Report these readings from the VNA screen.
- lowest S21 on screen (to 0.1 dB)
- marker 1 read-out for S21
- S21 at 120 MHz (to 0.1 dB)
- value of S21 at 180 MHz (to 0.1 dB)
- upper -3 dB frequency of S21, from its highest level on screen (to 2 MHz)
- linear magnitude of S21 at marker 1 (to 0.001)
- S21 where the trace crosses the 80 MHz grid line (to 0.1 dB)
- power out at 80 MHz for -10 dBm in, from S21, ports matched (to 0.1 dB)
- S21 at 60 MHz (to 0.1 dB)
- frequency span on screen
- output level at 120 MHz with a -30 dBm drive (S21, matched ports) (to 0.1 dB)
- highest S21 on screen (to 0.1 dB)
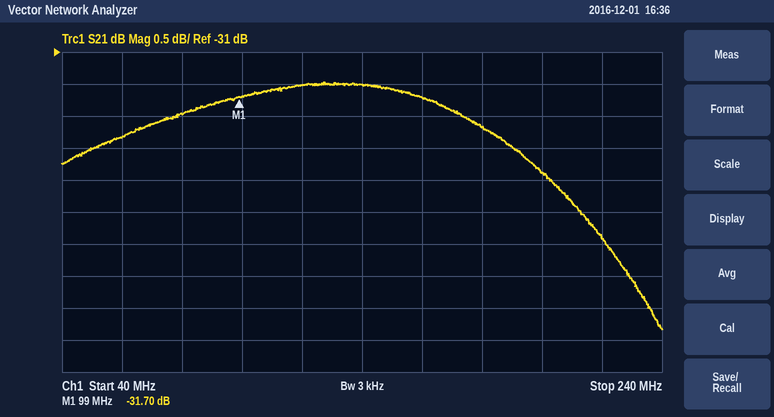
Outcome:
-35.3 dB
-31.70 dB
-31.5 dB
-32.2 dB
228 MHz
0.026
-32.0 dB
-42.0 dBm
-32.3 dB
200 MHz
-61.5 dBm
-31.5 dB
